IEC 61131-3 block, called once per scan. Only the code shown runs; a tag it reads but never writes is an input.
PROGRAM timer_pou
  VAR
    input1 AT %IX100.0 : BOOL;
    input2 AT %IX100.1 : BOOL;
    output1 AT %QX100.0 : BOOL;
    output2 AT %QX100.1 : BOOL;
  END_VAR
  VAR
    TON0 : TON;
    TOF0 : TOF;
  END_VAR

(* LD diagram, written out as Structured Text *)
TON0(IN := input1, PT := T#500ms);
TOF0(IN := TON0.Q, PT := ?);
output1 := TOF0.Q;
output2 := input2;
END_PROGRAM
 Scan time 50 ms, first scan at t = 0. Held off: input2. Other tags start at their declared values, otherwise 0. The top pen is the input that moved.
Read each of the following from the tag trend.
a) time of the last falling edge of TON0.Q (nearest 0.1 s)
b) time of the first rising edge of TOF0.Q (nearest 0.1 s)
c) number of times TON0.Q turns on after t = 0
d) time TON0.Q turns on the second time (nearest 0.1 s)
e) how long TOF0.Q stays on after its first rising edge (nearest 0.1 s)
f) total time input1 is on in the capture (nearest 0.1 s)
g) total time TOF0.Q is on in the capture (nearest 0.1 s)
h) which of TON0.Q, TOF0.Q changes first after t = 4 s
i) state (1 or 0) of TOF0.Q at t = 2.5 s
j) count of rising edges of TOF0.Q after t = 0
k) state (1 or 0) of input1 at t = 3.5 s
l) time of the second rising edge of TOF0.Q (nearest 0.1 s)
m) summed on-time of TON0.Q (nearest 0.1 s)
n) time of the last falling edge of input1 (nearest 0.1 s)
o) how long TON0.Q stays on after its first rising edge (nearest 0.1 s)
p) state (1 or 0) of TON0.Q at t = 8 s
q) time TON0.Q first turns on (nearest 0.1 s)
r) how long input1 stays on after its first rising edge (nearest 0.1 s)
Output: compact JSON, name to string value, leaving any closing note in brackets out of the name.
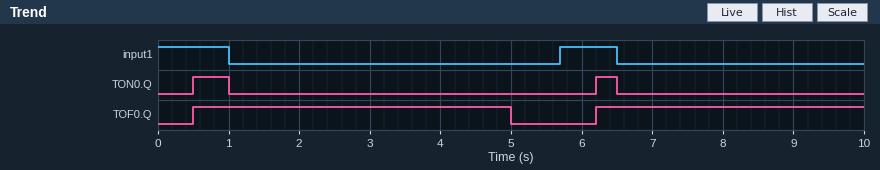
{"time of the last falling edge of TON0.Q": "6.5 s", "time of the first rising edge of TOF0.Q": "0.5 s", "number of times TON0.Q turns on after t = 0": "2", "time TON0.Q turns on the second time": "6.2 s", "how long TOF0.Q stays on after its first rising edge": "4.5 s", "total time input1 is on in the capture": "1.8 s", "total time TOF0.Q is on in the capture": "8.3 s", "which of TON0.Q, TOF0.Q changes first after t = 4 s": "TOF0.Q", "state (1 or 0) of TOF0.Q at t = 2.5 s": "1", "count of rising edges of TOF0.Q after t = 0": "2", "state (1 or 0) of input1 at t = 3.5 s": "0", "time of the second rising edge of TOF0.Q": "6.2 s", "summed on-time of TON0.Q": "0.8 s", "time of the last falling edge of input1": "6.5 s", "how long TON0.Q stays on after its first rising edge": "0.5 s", "state (1 or 0) of TON0.Q at t = 8 s": "0", "time TON0.Q first turns on": "0.5 s", "how long input1 stays on after its first rising edge": "0.8 s"}
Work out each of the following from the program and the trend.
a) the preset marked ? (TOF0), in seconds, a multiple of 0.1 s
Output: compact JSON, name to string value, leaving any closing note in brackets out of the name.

{"the preset marked ? (TOF0), in seconds, a multiple of 0.1 s": "4.0 s"}
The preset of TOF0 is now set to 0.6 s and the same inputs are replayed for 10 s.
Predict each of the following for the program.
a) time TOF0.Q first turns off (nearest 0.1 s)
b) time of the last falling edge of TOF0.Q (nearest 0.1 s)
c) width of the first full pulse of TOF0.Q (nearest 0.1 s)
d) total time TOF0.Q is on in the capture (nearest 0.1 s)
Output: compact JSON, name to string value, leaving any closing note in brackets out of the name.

{"time TOF0.Q first turns off": "1.6 s", "time of the last falling edge of TOF0.Q": "7.1 s", "width of the first full pulse of TOF0.Q": "1.1 s", "total time TOF0.Q is on in the capture": "2.0 s"}
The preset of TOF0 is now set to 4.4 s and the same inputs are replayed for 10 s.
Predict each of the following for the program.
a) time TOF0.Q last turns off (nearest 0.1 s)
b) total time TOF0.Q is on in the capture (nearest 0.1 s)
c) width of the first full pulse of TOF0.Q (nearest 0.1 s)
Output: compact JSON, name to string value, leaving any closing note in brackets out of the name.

{"time TOF0.Q last turns off": "5.4 s", "total time TOF0.Q is on in the capture": "8.7 s", "width of the first full pulse of TOF0.Q": "4.9 s"}
